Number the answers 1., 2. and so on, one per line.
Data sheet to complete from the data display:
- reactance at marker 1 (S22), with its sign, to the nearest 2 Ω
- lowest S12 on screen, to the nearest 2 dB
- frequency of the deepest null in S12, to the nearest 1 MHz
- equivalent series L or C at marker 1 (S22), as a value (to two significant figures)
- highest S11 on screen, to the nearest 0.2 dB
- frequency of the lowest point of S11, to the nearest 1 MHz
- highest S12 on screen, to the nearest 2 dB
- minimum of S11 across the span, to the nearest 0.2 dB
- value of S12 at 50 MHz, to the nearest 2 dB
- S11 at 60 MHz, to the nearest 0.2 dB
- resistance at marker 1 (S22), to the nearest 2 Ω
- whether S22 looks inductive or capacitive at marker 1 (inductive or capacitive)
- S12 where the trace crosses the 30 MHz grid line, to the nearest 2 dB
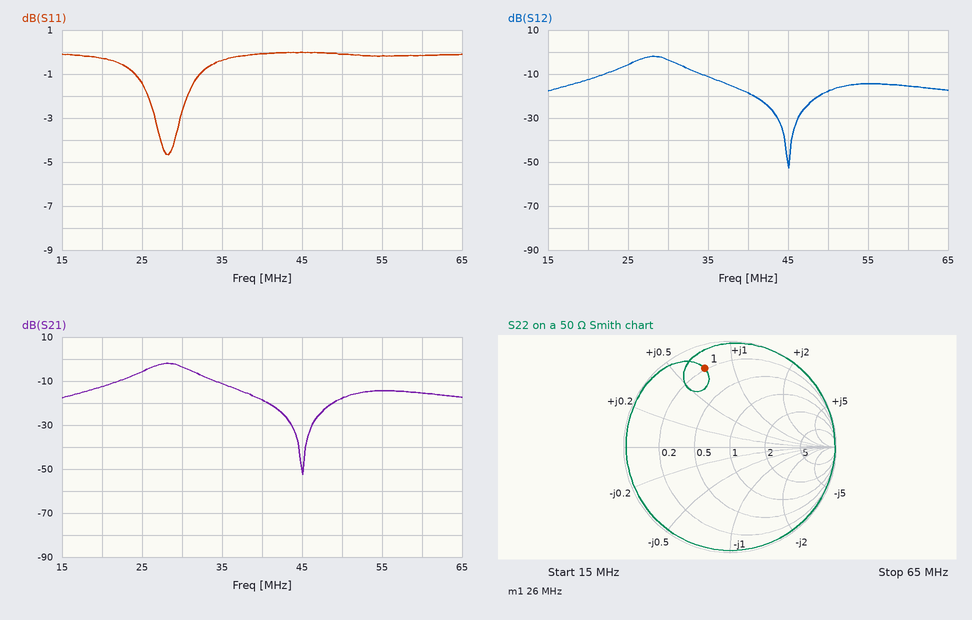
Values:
1. +36 Ω
2. -52 dB
3. 45 MHz
4. 220 nH
5. 0.0 dB
6. 28 MHz
7. -2 dB
8. -4.6 dB
9. -18 dB
10. -0.2 dB
11. 10 Ω
12. inductive
13. -4 dB
